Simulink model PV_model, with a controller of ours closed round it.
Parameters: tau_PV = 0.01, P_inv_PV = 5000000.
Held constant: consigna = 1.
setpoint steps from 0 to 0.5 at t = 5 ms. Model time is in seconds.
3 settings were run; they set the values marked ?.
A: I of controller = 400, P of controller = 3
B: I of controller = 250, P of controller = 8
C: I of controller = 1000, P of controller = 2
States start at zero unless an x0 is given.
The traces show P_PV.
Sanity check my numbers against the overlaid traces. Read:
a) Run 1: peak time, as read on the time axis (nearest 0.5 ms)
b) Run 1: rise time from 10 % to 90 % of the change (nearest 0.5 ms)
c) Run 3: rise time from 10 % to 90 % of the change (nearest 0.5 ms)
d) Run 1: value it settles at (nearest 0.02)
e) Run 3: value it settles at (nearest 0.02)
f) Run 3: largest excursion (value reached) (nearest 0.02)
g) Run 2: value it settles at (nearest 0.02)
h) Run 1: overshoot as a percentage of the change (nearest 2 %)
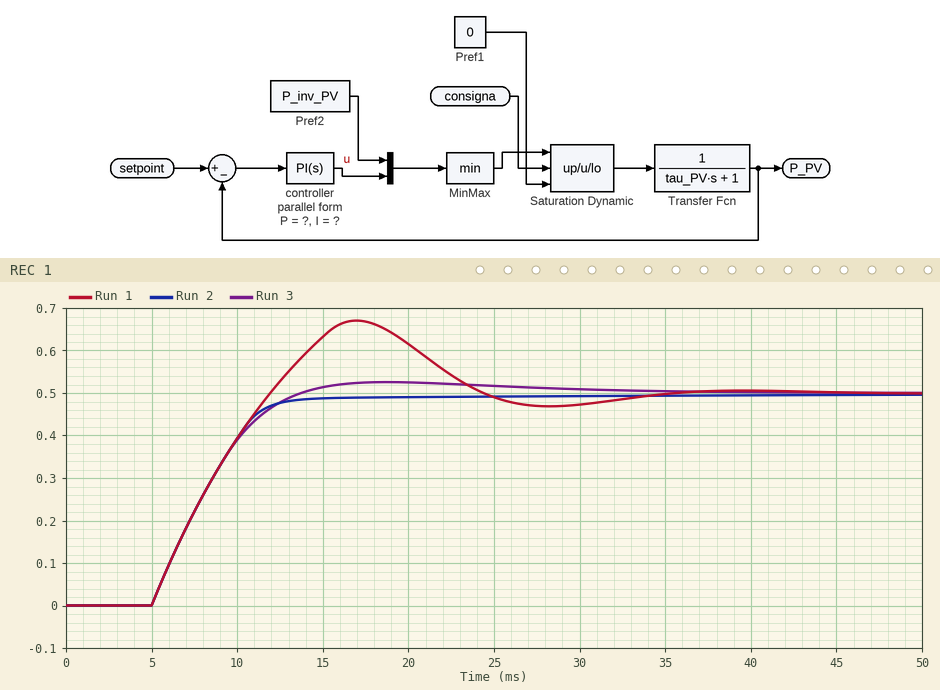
17.0 ms
5.5 ms
6.0 ms
0.50
0.50
0.52
0.50
34 %
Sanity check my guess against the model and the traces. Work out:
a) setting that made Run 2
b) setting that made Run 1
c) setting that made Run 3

B
C
A
